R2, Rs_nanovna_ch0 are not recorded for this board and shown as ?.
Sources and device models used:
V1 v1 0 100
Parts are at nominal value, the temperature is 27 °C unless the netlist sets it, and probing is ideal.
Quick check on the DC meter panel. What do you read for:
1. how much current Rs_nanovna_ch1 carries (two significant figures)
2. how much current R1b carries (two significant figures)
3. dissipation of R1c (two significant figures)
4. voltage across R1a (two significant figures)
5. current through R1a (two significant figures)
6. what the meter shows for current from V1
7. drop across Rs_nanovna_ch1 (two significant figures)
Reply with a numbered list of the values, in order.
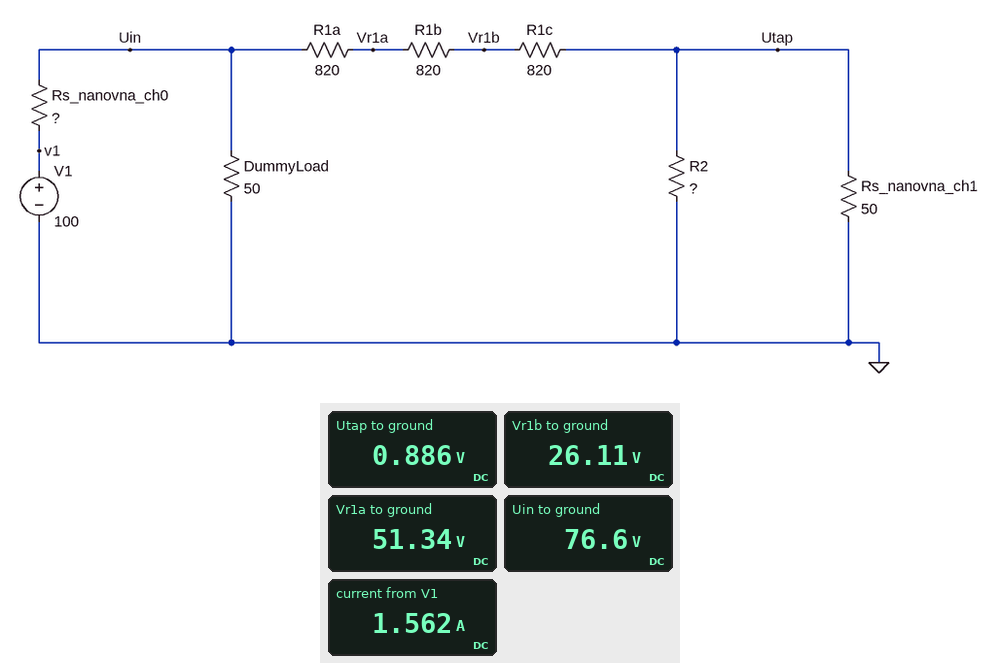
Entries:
1. 18 mA
2. 31 mA
3. 780 mW
4. 25 V
5. 31 mA
6. 1.562 A
7. 890 mV
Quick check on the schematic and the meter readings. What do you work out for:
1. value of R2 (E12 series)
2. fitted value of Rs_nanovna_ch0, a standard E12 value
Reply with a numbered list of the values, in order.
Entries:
1. 68 Ω
2. 15 Ω
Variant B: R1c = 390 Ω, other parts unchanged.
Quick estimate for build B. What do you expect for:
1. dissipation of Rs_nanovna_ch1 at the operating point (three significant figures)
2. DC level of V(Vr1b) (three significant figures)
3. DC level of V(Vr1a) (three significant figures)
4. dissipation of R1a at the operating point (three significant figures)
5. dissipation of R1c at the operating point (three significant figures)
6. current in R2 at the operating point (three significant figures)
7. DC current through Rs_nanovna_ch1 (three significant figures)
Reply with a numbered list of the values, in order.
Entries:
1. 22.9 mW
2. 15.6 V
3. 46.0 V
4. 1.13 W
5. 538 mW
6. 15.7 mA
7. 21.4 mA
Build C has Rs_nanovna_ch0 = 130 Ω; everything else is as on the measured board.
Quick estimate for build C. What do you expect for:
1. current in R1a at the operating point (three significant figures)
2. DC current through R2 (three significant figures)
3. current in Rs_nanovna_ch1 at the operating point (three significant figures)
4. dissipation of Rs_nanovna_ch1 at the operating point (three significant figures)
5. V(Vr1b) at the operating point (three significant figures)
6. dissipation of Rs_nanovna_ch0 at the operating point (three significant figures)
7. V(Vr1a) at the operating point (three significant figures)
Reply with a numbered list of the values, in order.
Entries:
1. 11.0 mA
2. 4.66 mA
3. 6.34 mA
4. 2.01 mW
5. 9.34 V
6. 40.6 W
7. 18.4 V
